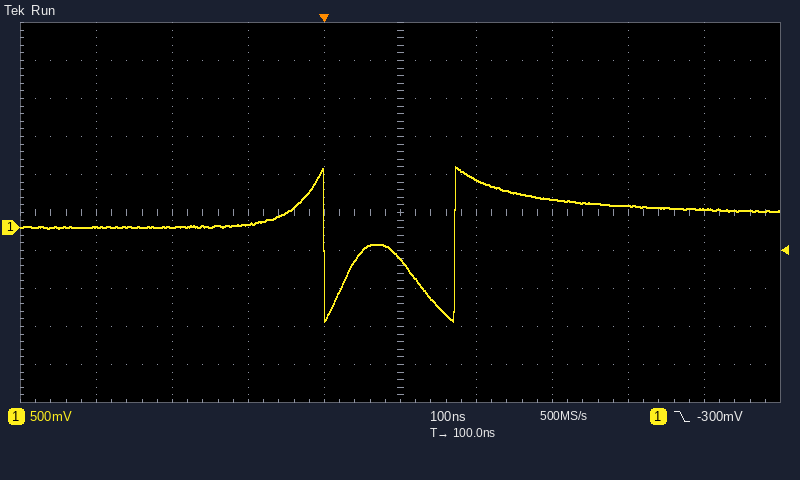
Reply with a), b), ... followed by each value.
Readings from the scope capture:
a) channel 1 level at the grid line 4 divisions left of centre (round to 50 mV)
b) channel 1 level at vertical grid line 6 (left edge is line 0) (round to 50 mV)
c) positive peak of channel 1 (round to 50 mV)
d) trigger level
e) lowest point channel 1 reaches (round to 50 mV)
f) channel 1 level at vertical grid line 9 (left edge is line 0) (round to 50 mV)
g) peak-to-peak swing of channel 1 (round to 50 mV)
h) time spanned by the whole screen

a) 0 mV
b) 650 mV
c) 800 mV
d) -300 mV
e) -1.25 V
f) 250 mV
g) 2.05 V
h) 1 µs
